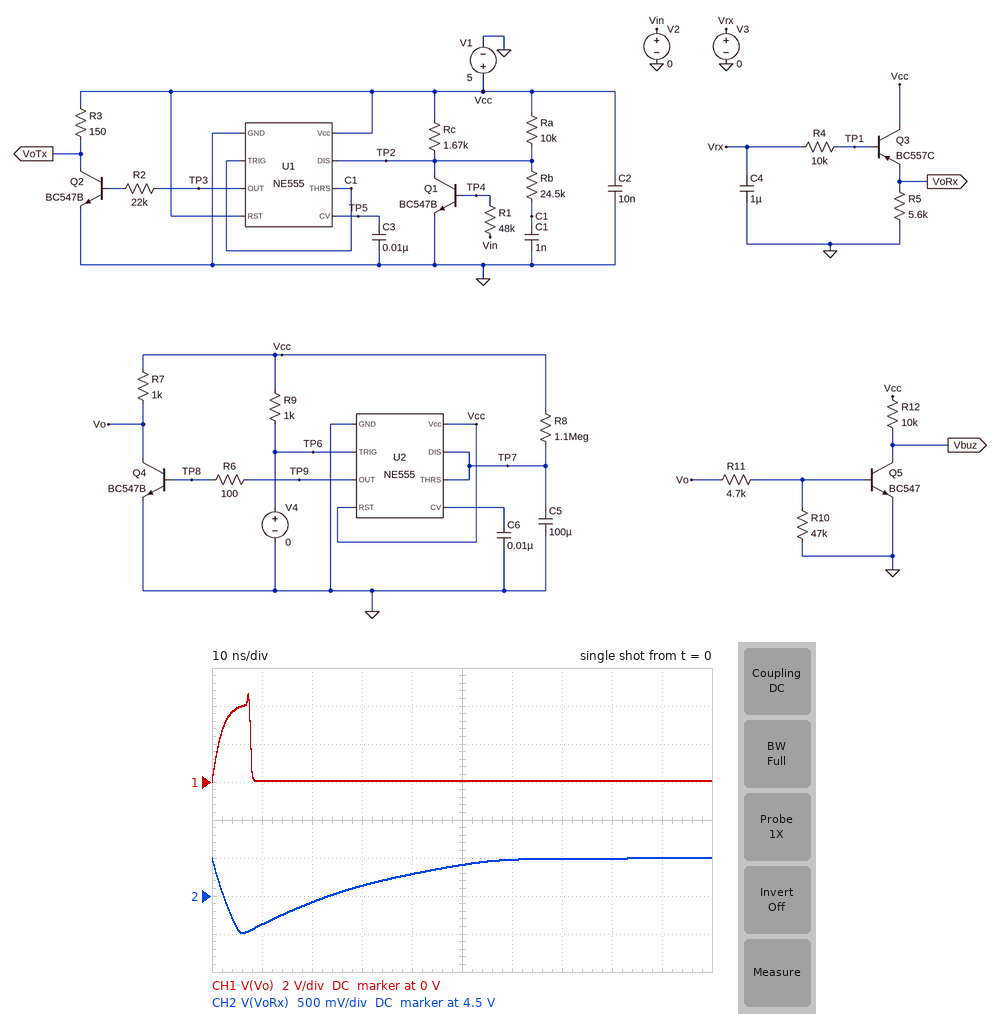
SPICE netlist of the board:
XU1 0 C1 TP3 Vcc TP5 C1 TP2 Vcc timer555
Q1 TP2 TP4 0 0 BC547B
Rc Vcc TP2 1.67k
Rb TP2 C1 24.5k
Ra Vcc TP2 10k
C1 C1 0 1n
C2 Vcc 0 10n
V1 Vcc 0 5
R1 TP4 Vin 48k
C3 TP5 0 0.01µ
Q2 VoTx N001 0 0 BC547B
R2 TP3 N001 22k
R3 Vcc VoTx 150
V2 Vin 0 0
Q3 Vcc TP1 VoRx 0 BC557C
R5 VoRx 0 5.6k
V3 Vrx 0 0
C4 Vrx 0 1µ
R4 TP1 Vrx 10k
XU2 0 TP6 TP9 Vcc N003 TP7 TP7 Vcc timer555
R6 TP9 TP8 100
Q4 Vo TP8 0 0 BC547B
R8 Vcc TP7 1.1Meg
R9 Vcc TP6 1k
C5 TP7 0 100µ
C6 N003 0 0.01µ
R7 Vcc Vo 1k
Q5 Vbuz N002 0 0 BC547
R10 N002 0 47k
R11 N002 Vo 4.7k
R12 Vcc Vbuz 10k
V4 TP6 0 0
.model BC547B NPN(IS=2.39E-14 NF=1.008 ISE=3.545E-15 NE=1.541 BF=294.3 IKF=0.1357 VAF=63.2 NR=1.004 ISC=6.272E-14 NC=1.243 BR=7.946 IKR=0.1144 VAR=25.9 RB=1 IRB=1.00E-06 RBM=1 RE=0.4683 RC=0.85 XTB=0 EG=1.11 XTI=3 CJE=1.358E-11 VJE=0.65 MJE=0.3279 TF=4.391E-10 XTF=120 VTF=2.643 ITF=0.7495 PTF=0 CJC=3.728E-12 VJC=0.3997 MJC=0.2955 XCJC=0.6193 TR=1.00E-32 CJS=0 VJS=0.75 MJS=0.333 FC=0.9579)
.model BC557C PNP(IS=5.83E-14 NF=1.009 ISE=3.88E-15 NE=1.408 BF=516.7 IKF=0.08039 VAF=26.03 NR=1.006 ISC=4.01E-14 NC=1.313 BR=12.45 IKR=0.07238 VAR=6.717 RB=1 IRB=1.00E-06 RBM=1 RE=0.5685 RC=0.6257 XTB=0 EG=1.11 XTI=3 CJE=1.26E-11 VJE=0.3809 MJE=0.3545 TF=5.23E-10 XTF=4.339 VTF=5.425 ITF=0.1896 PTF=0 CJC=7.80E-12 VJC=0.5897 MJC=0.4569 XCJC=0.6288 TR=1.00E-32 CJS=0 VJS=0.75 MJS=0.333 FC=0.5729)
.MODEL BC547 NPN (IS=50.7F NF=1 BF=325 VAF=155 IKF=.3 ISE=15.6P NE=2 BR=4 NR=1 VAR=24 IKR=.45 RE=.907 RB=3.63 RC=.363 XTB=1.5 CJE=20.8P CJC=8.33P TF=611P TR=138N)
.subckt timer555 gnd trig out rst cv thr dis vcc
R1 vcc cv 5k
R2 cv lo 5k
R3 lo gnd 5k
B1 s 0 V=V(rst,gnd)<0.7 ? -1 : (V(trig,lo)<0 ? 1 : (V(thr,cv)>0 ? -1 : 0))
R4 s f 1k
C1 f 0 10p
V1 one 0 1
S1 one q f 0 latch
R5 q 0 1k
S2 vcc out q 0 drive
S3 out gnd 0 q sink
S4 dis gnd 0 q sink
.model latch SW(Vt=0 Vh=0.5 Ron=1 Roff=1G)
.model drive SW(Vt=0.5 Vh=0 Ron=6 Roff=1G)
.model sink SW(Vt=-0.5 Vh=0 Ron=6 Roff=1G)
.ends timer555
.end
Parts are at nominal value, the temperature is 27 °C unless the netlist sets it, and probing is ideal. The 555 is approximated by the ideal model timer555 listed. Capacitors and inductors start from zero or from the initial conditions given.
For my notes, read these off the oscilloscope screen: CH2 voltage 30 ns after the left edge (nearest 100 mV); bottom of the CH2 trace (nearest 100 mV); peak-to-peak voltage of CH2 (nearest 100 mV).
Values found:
4.6 V
4.0 V
1.0 V
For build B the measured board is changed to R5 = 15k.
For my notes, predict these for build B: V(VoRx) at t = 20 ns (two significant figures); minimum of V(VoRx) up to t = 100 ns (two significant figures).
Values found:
4.5 V
4.2 V
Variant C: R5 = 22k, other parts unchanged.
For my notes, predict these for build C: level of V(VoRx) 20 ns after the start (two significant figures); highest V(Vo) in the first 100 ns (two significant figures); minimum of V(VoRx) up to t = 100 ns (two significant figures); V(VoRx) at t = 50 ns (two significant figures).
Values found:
4.5 V
4.6 V
4.3 V
5.0 V
